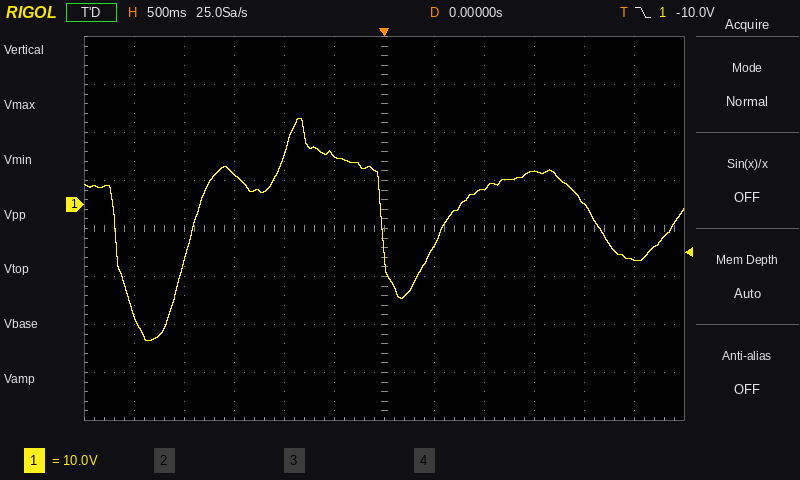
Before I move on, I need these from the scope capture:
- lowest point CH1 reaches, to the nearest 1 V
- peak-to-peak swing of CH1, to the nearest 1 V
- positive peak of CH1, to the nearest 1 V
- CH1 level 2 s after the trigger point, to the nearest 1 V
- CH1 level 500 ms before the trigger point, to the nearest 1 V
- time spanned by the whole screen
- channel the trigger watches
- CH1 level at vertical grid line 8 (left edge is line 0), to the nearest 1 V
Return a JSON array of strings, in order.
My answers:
["-28 V", "46 V", "18 V", "0 V", "10 V", "6 s", "CH1", "3 V"]
